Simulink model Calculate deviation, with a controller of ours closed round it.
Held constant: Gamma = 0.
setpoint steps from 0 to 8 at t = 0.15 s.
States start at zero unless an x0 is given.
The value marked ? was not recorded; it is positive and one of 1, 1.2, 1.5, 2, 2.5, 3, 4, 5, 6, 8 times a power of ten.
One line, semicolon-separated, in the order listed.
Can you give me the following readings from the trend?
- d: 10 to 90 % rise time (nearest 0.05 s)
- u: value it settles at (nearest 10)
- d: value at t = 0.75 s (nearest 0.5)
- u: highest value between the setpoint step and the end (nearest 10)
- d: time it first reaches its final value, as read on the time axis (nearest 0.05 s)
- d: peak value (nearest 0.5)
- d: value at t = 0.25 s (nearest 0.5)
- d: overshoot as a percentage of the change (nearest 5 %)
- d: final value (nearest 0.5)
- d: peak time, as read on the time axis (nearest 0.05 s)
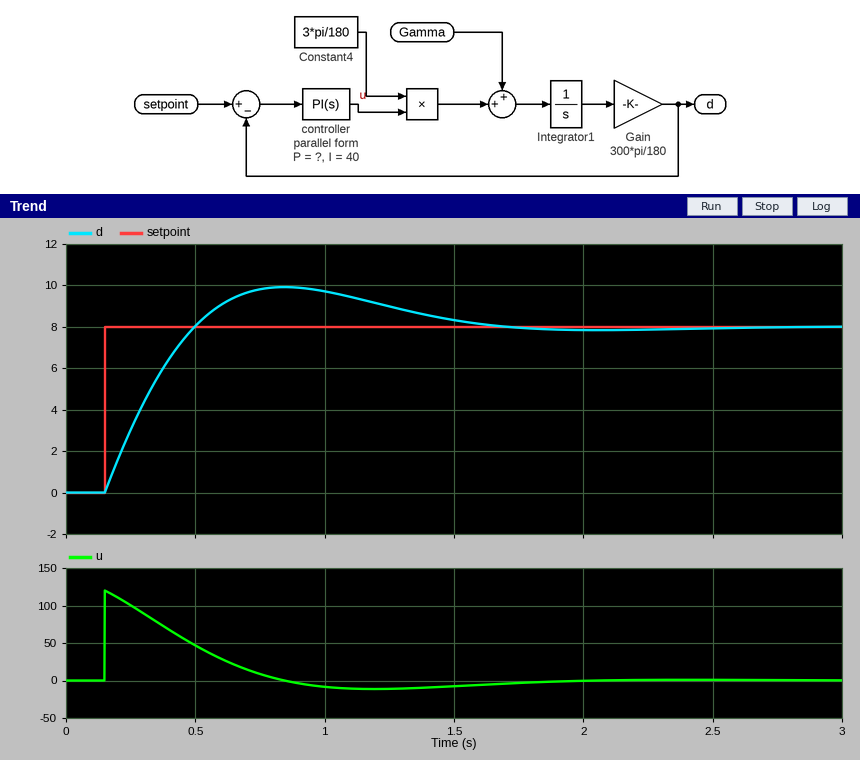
0.25 s; 0; 10.0; 120; 0.50 s; 10.0; 3.0; 25 %; 8.0; 0.85 s
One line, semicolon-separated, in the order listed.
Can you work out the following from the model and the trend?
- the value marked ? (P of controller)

15
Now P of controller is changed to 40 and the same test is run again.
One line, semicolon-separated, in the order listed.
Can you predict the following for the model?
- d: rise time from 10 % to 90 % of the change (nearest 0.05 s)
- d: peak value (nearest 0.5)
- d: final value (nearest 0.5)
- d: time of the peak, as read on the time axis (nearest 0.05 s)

0.15 s; 8.5; 8.0; 0.65 s
